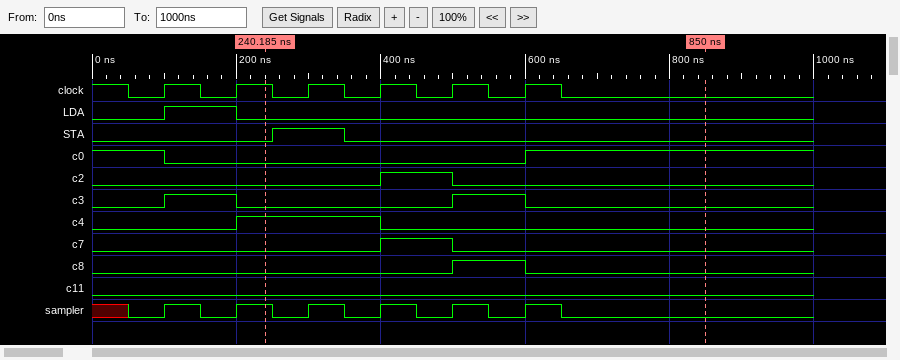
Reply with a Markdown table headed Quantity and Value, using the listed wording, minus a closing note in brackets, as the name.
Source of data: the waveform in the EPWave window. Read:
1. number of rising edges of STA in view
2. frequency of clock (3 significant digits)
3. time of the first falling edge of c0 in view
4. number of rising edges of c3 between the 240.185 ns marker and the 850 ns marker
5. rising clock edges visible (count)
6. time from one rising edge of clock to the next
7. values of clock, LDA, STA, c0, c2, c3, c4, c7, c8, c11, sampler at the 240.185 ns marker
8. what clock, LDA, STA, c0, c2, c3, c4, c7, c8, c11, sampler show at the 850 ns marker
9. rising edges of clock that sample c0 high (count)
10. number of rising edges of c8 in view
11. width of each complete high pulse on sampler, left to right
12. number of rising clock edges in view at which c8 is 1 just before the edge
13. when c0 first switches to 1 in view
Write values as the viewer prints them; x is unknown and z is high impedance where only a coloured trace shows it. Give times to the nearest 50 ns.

| Quantity | Value |
|---|---|
| number of rising edges of STA in view | 1 |
| frequency of clock | 10.0 MHz |
| time of the first falling edge of c0 in view | 100 ns |
| number of rising edges of c3 between the 240.185 ns marker and the 850 ns marker | 1 |
| rising clock edges visible | 6 |
| time from one rising edge of clock to the next | 100 ns |
| values of clock, LDA, STA, c0, c2, c3, c4, c7, c8, c11, sampler at the 240.185 ns marker | clock=1, LDA=0, STA=0, c0=0, c2=0, c3=0, c4=1, c7=0, c8=0, c11=0, sampler=1 |
| what clock, LDA, STA, c0, c2, c3, c4, c7, c8, c11, sampler show at the 850 ns marker | clock=0, LDA=0, STA=0, c0=1, c2=0, c3=0, c4=0, c7=0, c8=0, c11=0, sampler=0 |
| rising edges of clock that sample c0 high | 1 |
| number of rising edges of c8 in view | 1 |
| width of each complete high pulse on sampler, left to right | 50 ns, 50 ns, 50 ns, 50 ns, 50 ns, 50 ns |
| number of rising clock edges in view at which c8 is 1 just before the edge | 1 |
| when c0 first switches to 1 in view | 600 ns |
